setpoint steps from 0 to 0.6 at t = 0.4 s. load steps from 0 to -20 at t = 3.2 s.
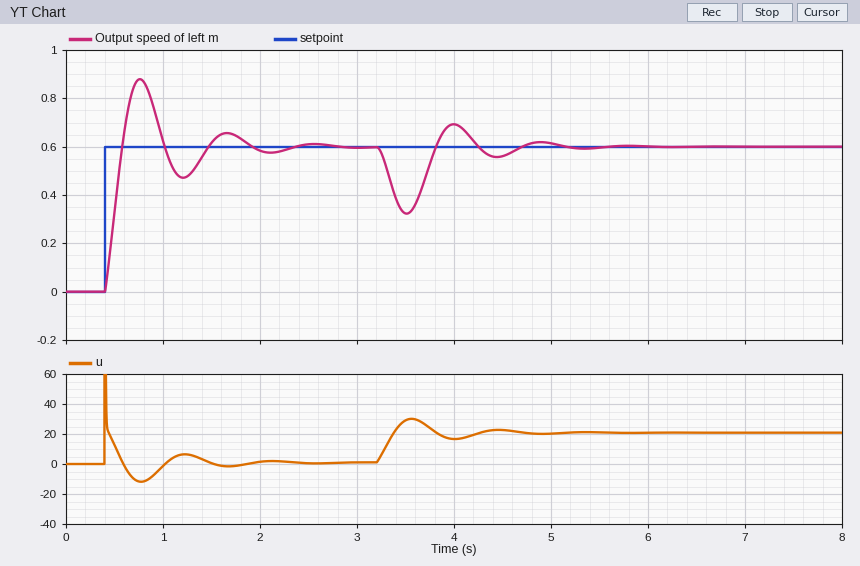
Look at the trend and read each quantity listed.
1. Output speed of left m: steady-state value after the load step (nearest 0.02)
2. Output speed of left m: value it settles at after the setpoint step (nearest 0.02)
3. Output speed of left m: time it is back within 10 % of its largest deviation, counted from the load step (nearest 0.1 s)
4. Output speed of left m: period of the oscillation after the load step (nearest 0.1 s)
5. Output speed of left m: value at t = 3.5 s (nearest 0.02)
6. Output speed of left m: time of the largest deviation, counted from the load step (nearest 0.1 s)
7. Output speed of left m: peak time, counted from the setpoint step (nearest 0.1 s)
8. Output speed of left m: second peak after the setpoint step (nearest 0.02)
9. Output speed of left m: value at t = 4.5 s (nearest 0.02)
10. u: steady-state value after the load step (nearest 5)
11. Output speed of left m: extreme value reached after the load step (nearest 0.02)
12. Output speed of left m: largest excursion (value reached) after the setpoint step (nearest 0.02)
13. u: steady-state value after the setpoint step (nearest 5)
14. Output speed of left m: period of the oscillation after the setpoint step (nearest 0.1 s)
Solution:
0.60
0.60
1.4 s
0.9 s
0.32
0.3 s
0.4 s
0.66
0.56
20
0.32
0.88
0
0.9 s
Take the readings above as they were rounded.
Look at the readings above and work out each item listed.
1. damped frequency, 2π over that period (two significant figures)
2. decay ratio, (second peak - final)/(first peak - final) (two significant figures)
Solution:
7.0 rad/s
0.21
